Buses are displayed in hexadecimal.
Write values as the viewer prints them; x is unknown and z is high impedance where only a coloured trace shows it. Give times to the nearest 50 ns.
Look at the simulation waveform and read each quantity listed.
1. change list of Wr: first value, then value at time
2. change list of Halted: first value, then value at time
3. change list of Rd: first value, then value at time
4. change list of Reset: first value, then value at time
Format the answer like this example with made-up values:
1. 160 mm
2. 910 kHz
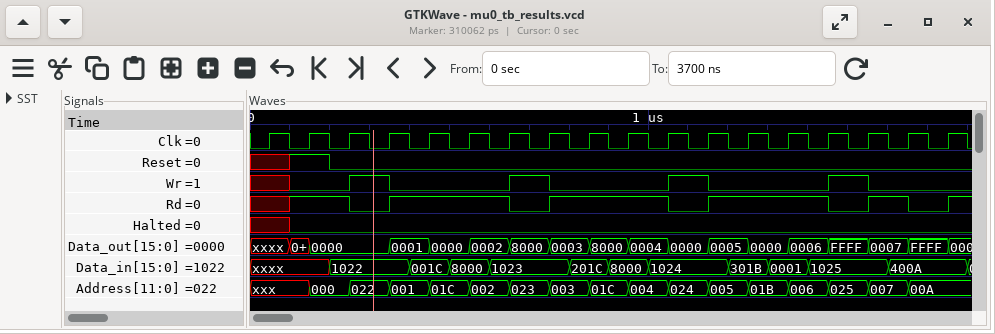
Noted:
1. x, 0 at 100 ns, 1 at 250 ns, 0 at 350 ns, 1 at 650 ns, 0 at 750 ns, 1 at 1050 ns, 0 at 1150 ns, 1 at 1450 ns, 0 at 1550 ns
2. x, 0 at 100 ns
3. x, 1 at 100 ns, 0 at 250 ns, 1 at 350 ns, 0 at 650 ns, 1 at 750 ns, 0 at 1050 ns, 1 at 1150 ns, 0 at 1450 ns, 1 at 1550 ns, 0 at 1650 ns, 1 at 1750 ns
4. x, 1 at 100 ns, 0 at 200 ns
